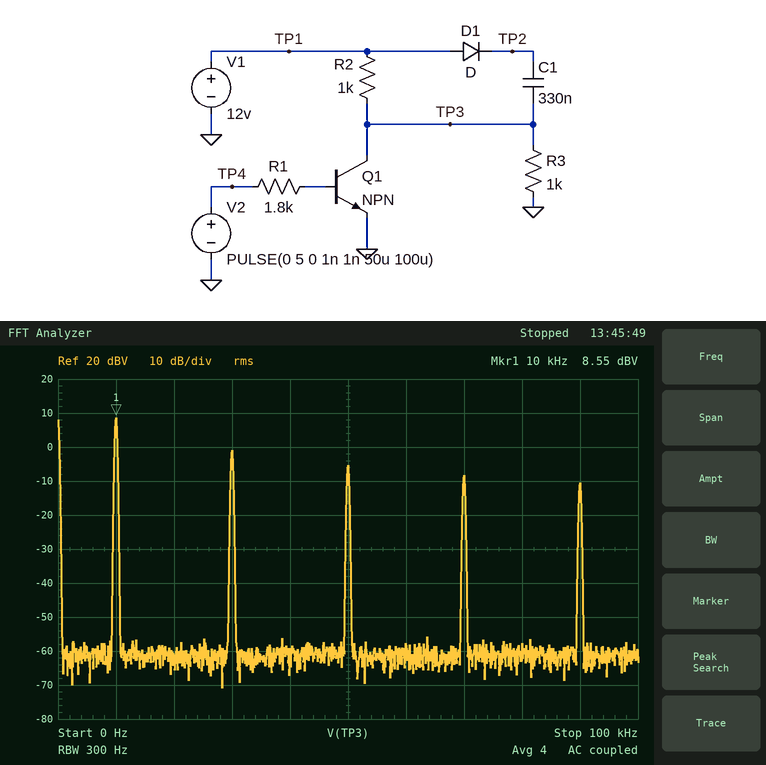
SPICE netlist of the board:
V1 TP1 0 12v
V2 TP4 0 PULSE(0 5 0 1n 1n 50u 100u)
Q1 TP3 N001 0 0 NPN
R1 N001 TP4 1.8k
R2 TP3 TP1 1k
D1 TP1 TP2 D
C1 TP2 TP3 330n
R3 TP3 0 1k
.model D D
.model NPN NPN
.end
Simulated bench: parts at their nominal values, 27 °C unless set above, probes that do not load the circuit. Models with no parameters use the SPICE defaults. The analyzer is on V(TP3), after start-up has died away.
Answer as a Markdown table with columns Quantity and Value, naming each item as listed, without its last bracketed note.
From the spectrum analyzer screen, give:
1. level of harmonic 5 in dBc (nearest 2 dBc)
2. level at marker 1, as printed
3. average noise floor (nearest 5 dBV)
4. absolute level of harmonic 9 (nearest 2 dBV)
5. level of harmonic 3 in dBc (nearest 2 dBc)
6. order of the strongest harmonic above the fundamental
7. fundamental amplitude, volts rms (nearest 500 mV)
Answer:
| Quantity | Value |
|---|---|
| level of harmonic 5 in dBc | -14 dBc |
| level at marker 1, as printed | 8.55 dBV |
| average noise floor | -60 dBV |
| absolute level of harmonic 9 | -10 dBV |
| level of harmonic 3 in dBc | -10 dBc |
| order of the strongest harmonic above the fundamental | 3 |
| fundamental amplitude, volts rms | 2.5 V |
